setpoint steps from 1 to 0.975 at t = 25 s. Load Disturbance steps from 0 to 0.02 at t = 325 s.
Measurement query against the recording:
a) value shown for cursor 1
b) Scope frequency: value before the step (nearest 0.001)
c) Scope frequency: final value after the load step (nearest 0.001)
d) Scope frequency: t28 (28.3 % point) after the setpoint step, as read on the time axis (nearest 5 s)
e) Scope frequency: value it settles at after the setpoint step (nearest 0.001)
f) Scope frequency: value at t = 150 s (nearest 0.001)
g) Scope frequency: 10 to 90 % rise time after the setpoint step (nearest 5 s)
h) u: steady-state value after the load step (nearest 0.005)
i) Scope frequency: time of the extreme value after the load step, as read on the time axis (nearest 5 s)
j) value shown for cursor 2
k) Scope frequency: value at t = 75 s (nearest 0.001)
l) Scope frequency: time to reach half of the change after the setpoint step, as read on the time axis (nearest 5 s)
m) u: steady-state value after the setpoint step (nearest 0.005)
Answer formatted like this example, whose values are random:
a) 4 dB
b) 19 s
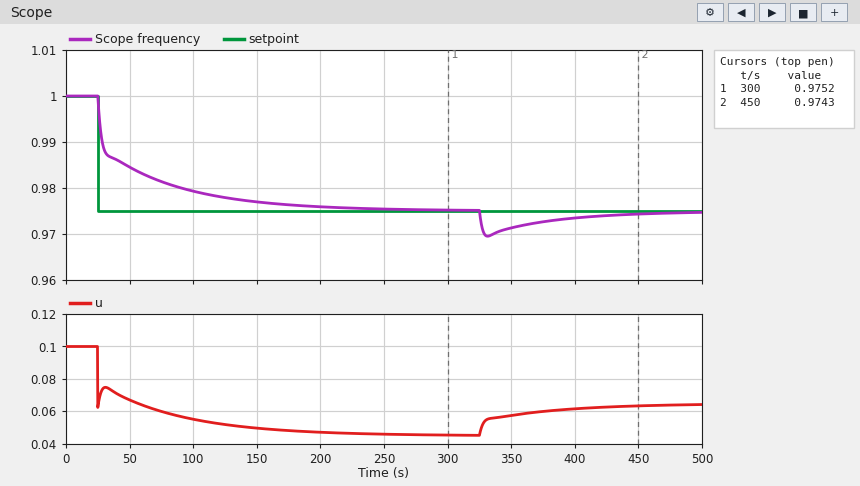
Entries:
a) 0.9752
b) 1.000
c) 0.975
d) 25 s
e) 0.975
f) 0.977
g) 110 s
h) 0.065
i) 330 s
j) 0.9743
k) 0.981
l) 30 s
m) 0.045
